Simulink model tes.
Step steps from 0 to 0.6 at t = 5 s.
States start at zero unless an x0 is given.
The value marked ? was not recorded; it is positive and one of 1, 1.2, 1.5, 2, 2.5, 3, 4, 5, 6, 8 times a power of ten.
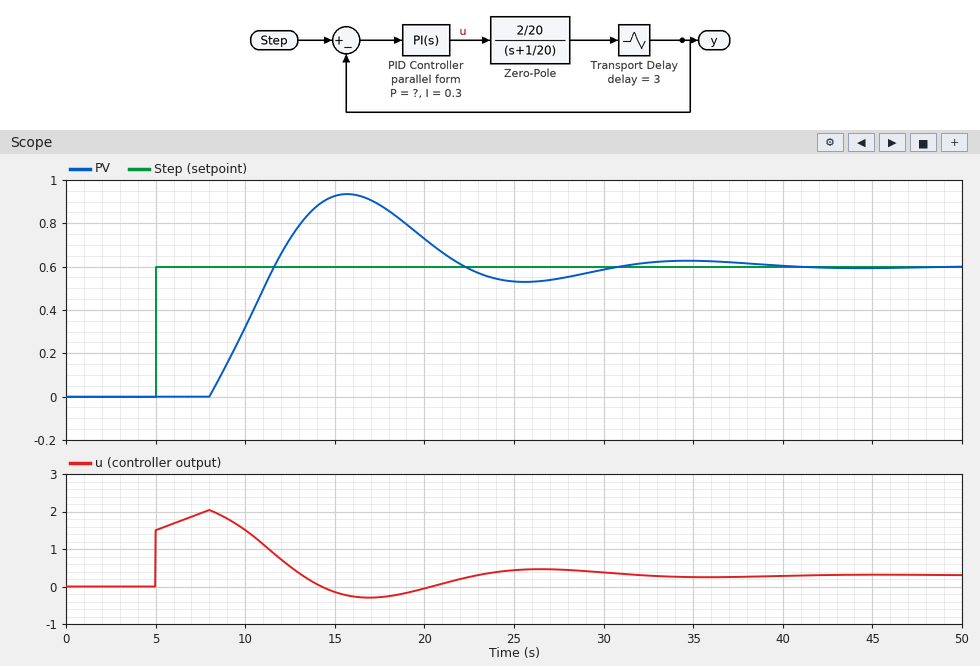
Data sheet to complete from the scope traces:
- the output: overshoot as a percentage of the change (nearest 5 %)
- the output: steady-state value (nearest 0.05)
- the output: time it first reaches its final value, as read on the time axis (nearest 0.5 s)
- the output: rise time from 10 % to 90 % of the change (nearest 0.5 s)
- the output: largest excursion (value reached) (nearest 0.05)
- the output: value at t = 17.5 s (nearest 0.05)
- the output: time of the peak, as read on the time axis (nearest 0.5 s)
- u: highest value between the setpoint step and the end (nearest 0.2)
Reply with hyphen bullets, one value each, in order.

- 55 %
- 0.60
- 11.5 s
- 3.0 s
- 0.95
- 0.90
- 15.5 s
- 2.0
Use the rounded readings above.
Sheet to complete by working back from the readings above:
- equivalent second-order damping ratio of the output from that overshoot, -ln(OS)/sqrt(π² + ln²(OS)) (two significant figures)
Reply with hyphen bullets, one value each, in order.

- 0.19
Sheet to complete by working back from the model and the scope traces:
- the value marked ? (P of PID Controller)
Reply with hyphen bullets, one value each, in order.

- 2.5
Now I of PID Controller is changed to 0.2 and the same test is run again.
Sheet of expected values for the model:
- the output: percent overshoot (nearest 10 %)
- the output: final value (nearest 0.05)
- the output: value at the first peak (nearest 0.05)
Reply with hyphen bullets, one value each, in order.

- 40 %
- 0.60
- 0.85
